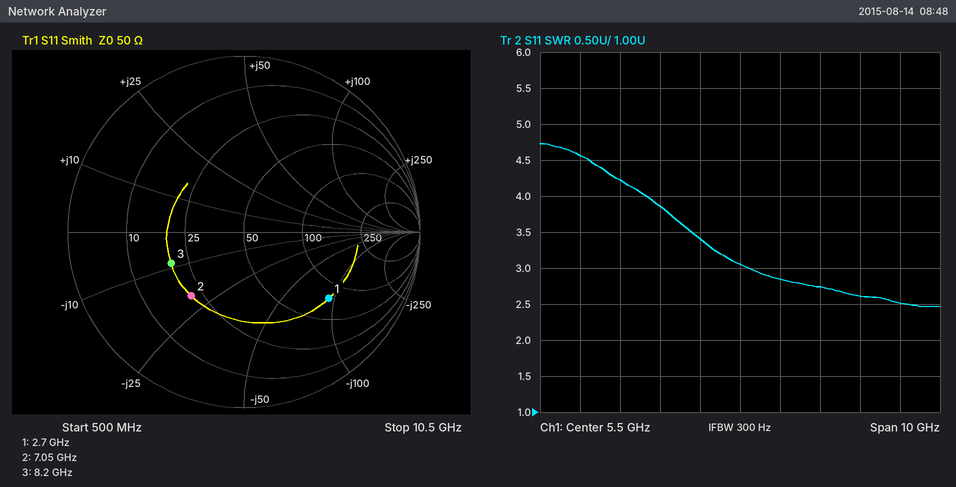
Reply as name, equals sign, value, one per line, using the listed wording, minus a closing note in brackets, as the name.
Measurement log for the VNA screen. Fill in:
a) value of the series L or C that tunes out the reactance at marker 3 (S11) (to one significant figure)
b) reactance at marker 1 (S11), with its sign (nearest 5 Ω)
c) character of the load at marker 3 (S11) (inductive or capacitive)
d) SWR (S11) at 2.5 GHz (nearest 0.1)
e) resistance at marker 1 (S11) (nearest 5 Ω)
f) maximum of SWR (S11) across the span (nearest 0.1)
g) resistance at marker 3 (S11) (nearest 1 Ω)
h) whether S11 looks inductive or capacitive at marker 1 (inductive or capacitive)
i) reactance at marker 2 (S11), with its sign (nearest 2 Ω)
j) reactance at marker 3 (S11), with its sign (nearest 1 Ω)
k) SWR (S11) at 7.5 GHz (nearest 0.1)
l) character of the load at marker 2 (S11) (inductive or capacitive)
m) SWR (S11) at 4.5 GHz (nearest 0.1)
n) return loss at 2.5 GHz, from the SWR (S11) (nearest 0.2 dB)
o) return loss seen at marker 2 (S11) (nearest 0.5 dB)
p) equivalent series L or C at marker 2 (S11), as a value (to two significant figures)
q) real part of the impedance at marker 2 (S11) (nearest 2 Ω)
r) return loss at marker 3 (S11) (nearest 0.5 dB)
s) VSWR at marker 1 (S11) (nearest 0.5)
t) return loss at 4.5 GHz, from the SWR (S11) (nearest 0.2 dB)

value of the series L or C that tunes out the reactance at marker 3 (S11) = 200 pH
reactance at marker 1 (S11), with its sign = -90 Ω
character of the load at marker 3 (S11) = capacitive
SWR (S11) at 2.5 GHz = 4.2
resistance at marker 1 (S11) = 75 Ω
maximum of SWR (S11) across the span = 4.7
resistance at marker 3 (S11) = 20 Ω
whether S11 looks inductive or capacitive at marker 1 = capacitive
reactance at marker 2 (S11), with its sign = -20 Ω
reactance at marker 3 (S11), with its sign = -9 Ω
SWR (S11) at 7.5 GHz = 2.7
character of the load at marker 2 (S11) = capacitive
SWR (S11) at 4.5 GHz = 3.4
return loss at 2.5 GHz, from the SWR (S11) = 4.2 dB
return loss seen at marker 2 (S11) = 6.5 dB
equivalent series L or C at marker 2 (S11), as a value = 1.1 pF
real part of the impedance at marker 2 (S11) = 22 Ω
return loss at marker 3 (S11) = 7.0 dB
VSWR at marker 1 (S11) = 4.0
return loss at 4.5 GHz, from the SWR (S11) = 5.2 dB
